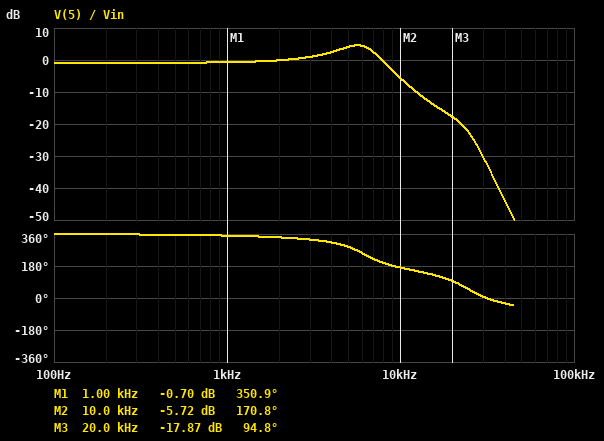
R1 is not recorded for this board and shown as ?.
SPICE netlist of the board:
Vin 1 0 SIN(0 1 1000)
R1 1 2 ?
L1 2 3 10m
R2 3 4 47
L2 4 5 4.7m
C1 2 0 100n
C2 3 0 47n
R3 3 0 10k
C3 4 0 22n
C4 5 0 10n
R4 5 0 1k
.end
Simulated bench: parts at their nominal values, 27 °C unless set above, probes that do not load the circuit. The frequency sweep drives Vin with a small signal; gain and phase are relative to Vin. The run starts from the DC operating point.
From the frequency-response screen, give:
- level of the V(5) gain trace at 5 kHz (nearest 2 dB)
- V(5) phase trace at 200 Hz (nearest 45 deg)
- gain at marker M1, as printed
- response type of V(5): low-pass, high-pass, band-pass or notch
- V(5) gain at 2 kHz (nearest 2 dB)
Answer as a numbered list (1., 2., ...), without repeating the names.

1. 4 dB
2. 360 deg
3. -0.70 dB
4. low-pass
5. 0 dB
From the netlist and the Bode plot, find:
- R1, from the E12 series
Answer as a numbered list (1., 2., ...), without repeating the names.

1. 56 Ω
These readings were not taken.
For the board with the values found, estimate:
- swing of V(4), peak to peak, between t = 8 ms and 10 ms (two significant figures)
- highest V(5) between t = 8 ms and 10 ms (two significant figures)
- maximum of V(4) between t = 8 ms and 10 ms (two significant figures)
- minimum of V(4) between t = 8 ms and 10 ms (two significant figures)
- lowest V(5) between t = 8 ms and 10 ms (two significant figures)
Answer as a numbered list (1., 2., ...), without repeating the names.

1. 1.8 V
2. 920 mV
3. 920 mV
4. -920 mV
5. -920 mV
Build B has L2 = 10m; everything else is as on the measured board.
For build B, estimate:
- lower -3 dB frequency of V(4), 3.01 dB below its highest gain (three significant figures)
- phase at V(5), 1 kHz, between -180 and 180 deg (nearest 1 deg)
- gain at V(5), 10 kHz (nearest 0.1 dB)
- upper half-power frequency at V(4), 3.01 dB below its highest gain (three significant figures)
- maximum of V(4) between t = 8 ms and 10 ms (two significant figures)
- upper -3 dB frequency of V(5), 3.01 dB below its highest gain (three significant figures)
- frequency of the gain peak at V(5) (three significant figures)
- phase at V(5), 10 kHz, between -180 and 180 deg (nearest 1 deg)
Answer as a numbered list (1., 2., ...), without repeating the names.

1. 3.16 kHz
2. -11 deg
3. -4.3 dB
4. 7.57 kHz
5. 920 mV
6. 7.68 kHz
7. 5.87 kHz
8. 150 deg
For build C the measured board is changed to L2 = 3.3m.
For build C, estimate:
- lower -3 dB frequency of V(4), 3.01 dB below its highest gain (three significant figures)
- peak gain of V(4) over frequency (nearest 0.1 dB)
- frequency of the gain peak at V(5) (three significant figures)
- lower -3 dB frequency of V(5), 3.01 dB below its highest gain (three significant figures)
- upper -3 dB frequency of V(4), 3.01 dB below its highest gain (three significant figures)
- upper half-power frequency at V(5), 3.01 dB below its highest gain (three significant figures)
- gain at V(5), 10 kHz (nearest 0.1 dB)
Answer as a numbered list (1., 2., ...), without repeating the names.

1. 3.31 kHz
2. 4.3 dB
3. 5.62 kHz
4. 3.44 kHz
5. 7.13 kHz
6. 7.19 kHz
7. -6.2 dB
